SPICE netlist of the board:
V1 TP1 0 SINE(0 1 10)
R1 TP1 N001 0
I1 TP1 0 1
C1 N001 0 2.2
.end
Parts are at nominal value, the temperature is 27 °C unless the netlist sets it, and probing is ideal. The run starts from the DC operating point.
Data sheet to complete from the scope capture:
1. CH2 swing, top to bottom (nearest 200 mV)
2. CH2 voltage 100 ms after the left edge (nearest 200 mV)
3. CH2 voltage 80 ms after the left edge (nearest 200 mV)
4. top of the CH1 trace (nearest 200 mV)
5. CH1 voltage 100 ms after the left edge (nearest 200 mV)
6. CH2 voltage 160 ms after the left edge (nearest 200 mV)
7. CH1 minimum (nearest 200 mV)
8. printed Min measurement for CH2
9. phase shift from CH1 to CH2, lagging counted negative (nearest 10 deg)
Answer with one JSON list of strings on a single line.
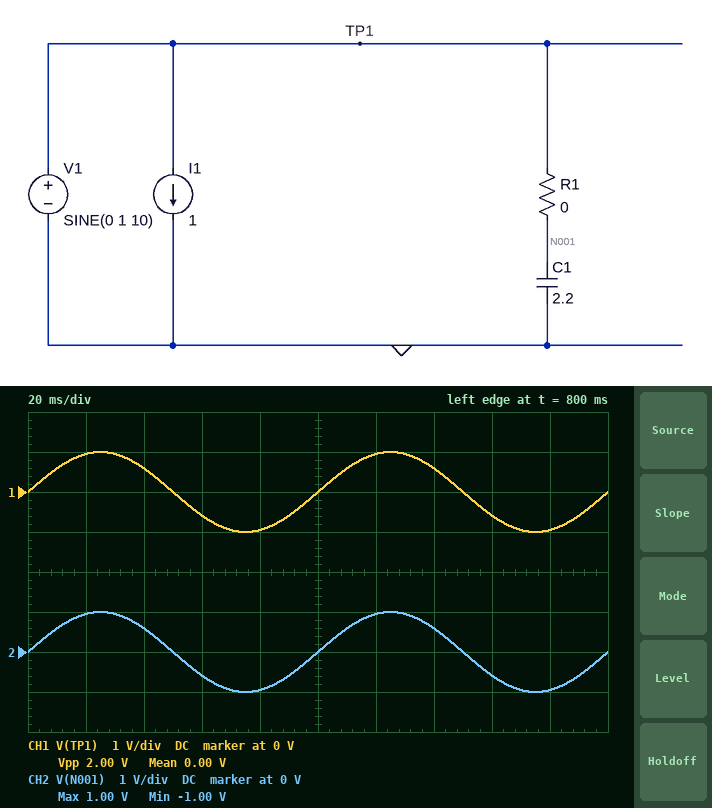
["2.0 V", "0 V", "-1.0 V", "1.0 V", "0 V", "-600 mV", "-1.0 V", "-1.00 V", "0 deg"]
